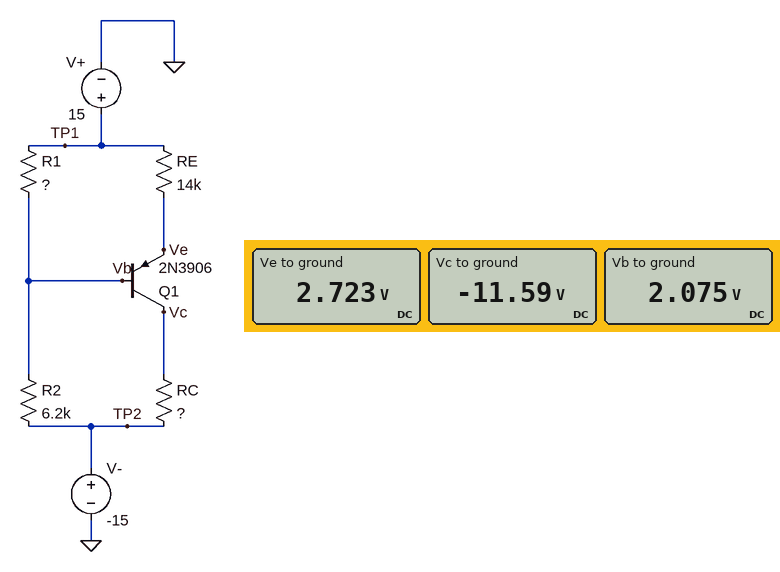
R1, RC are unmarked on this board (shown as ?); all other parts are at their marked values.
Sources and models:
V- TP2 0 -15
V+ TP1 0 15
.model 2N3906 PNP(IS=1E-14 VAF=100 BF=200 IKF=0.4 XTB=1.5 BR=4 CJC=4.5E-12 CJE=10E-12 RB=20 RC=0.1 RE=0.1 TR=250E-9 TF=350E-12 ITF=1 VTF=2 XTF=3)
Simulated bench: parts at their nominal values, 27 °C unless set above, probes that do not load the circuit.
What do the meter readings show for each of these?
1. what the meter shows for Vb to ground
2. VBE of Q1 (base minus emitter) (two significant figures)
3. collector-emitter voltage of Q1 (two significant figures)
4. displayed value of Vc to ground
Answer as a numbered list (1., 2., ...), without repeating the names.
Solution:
1. 2.075 V
2. -650 mV
3. -14 V
4. -11.59 V
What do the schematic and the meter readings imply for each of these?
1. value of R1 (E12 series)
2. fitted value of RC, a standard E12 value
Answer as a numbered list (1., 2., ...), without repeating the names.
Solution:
1. 4.7 kΩ
2. 3.9 kΩ
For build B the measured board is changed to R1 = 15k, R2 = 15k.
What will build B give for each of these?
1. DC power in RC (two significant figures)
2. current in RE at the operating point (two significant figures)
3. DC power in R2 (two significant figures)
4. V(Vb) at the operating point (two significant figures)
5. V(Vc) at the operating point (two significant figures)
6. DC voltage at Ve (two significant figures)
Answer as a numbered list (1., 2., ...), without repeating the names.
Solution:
1. 4.0 mW
2. 1.0 mA
3. 15 mW
4. 34 mV
5. -11 V
6. 690 mV
